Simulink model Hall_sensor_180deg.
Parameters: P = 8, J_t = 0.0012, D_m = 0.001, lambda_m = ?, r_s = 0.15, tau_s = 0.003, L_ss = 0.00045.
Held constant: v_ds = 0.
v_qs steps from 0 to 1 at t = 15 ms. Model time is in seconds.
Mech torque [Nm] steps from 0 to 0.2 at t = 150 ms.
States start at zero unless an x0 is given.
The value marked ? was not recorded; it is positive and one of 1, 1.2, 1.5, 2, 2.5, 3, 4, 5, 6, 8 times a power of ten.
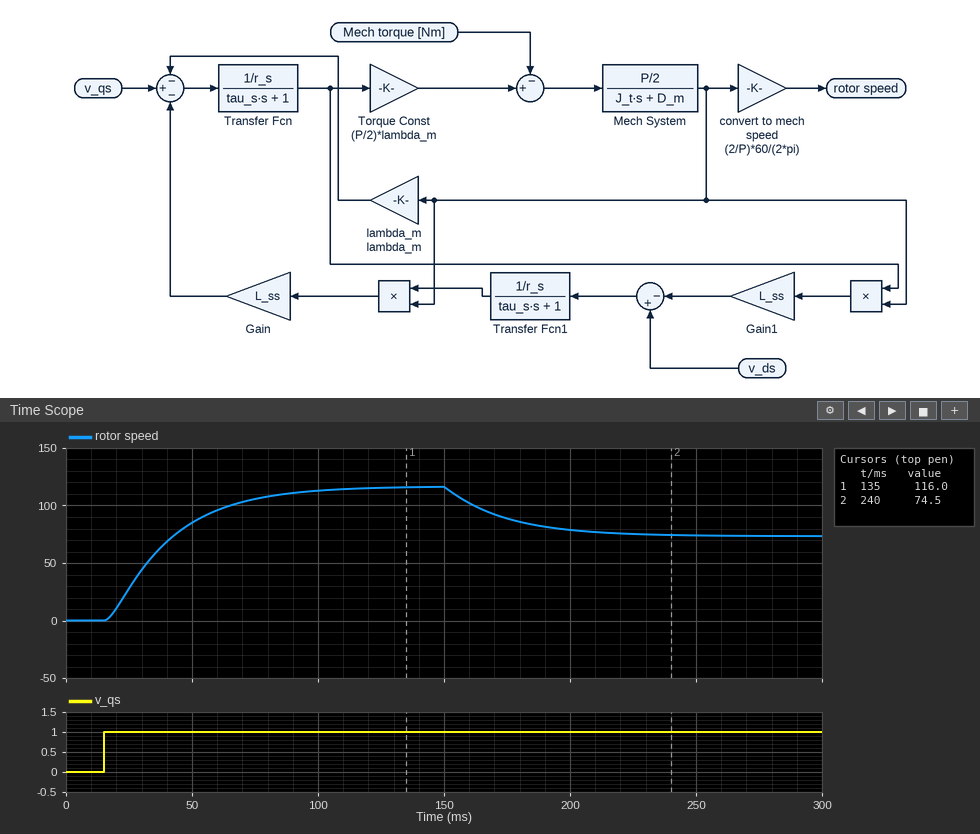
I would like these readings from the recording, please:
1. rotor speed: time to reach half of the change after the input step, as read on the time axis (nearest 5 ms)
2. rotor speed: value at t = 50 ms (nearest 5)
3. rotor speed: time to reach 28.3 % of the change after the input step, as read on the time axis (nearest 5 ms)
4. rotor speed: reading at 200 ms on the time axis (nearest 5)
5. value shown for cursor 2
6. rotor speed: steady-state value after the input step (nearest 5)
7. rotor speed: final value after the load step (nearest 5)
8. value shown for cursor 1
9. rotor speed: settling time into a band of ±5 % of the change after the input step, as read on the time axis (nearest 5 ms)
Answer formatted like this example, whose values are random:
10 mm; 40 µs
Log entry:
35 ms; 85; 25 ms; 80; 74.5; 115; 75; 116.0; 90 ms
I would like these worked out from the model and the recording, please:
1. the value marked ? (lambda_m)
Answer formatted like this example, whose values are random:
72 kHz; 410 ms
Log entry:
0.02
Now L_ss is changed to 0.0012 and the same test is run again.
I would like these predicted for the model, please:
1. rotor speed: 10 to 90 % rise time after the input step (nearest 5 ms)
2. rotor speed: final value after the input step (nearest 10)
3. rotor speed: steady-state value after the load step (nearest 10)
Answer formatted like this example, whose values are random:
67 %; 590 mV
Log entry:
50 ms; 120; 80
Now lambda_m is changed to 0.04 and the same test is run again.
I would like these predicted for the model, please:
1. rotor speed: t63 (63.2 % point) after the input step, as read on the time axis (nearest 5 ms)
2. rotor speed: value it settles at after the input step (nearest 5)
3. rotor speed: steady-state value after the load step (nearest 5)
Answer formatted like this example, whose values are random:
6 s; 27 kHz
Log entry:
25 ms; 60; 50
